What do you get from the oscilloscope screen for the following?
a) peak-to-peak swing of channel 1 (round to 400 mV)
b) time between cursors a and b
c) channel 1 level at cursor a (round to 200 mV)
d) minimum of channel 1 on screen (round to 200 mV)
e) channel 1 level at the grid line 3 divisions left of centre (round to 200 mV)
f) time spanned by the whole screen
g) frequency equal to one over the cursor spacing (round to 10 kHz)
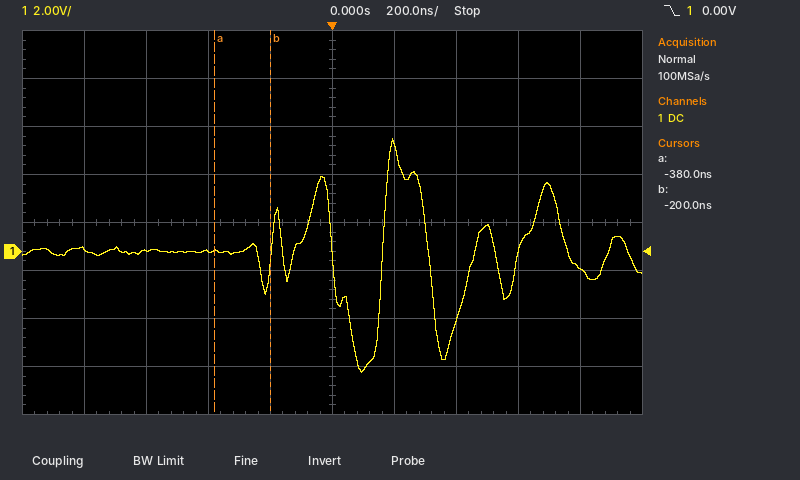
9.6 V
180 ns
0.0 V
-5.0 V
0.0 V
2 µs
5.56 MHz
